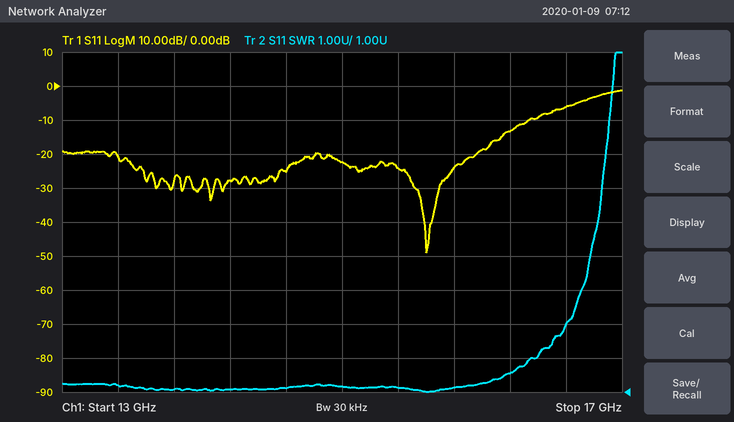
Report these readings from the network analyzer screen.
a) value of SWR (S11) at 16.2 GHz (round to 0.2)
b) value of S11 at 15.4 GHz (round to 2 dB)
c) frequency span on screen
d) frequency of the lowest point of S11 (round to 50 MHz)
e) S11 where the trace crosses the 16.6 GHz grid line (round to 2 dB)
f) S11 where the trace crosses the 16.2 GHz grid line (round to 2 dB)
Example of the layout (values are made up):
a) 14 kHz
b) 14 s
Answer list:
a) 1.6
b) -24 dB
c) 4 GHz
d) 15.60 GHz
e) -6 dB
f) -14 dB
